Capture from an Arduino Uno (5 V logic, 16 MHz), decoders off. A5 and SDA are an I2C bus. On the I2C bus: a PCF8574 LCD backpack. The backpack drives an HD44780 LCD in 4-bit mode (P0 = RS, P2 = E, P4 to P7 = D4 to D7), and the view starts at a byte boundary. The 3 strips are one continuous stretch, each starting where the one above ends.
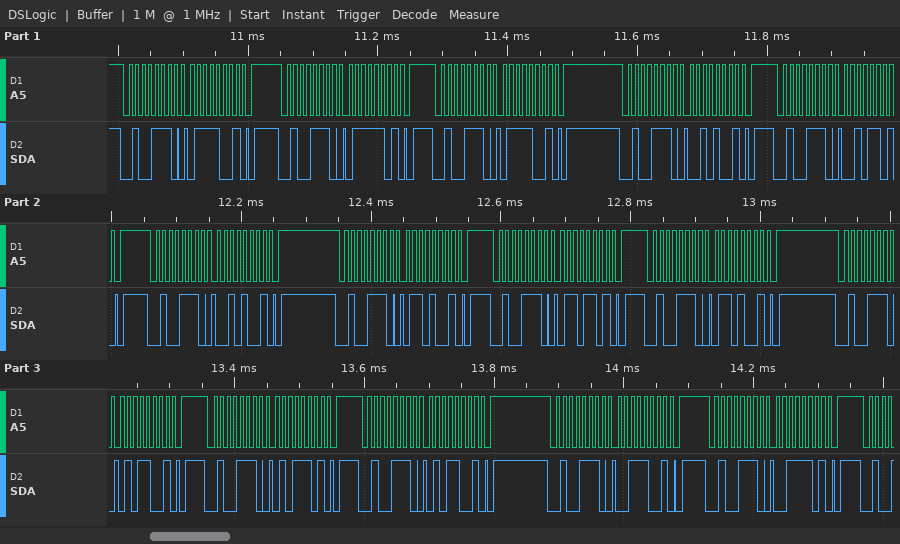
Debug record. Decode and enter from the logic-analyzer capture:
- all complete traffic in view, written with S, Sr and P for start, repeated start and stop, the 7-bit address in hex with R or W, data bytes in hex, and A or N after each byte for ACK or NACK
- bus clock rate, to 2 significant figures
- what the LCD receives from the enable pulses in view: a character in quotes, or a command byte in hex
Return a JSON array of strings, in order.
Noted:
["S 27W A 79 A P S 27W A 7D A P S 27W A 79 A P S 27W A 29 A P S 27W A 2D A P S 27W A 29 A P S 27W A 69 A P S 27W A 6D A P S 27W A 69 A P S 27W A 59 A P S 27W A 5D A P S 27W A 59 A P S 27W A 39 A P S 27W A 3D A P", "100 kHz", "'r' 'e'"]
